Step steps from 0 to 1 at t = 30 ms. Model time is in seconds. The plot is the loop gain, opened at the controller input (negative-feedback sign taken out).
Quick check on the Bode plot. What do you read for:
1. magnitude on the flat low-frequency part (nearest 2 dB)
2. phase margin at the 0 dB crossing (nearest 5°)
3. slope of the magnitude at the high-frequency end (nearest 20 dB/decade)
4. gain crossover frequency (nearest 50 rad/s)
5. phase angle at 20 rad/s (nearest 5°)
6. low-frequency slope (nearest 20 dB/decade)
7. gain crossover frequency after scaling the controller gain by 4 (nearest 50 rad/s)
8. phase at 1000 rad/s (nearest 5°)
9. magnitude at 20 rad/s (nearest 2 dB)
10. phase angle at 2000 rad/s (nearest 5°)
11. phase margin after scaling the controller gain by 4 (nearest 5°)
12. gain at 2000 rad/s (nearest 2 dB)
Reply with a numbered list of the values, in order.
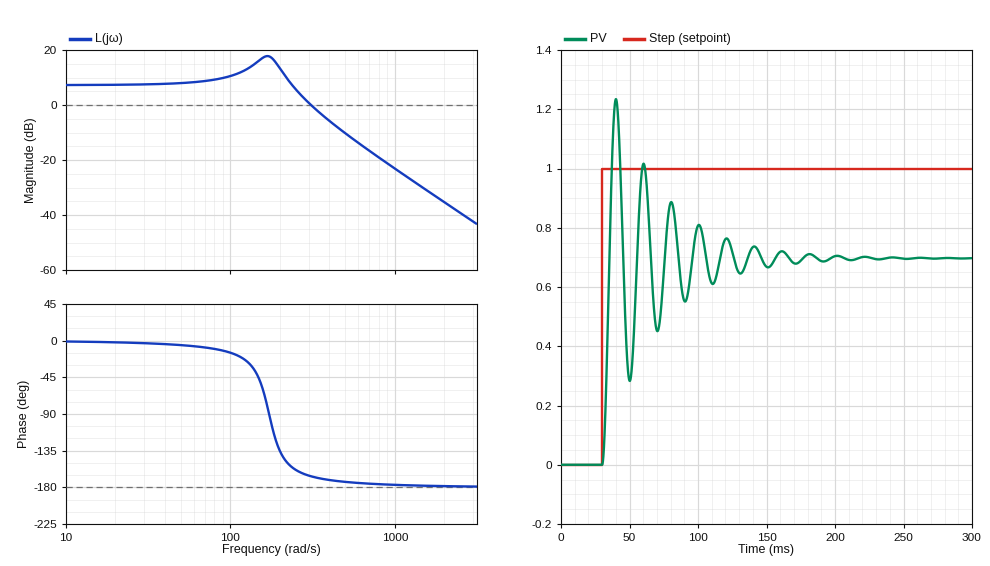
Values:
1. 8 dB
2. 15°
3. -40 dB/decade
4. 300 rad/s
5. 0°
6. 0 dB/decade
7. 550 rad/s
8. -175°
9. 8 dB
10. -180°
11. 5°
12. -36 dB
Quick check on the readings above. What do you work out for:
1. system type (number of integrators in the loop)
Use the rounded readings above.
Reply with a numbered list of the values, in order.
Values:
1. 0
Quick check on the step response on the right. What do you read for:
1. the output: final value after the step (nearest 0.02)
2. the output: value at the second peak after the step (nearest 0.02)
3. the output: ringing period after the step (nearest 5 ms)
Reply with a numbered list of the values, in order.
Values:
1. 0.70
2. 1.02
3. 20 ms
